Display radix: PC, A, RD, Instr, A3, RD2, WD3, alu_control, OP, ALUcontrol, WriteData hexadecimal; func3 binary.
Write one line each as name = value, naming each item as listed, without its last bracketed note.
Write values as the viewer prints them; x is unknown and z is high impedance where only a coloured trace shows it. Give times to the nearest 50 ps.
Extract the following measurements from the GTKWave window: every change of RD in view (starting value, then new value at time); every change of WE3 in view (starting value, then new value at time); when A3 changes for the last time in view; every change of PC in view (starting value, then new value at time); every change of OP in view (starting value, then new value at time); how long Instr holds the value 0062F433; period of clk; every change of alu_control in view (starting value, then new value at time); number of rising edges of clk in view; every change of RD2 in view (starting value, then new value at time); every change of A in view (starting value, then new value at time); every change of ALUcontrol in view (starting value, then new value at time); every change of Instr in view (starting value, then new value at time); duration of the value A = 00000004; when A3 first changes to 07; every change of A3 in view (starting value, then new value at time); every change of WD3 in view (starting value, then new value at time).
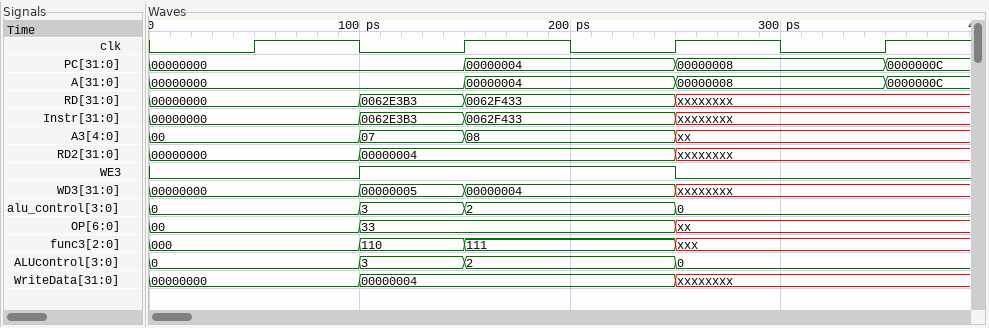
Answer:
every change of RD in view = 00000000, 0062E3B3 at 100 ps, 0062F433 at 150 ps, xxxxxxxx at 250 ps
every change of WE3 in view = 0, 1 at 100 ps, 0 at 250 ps
when A3 changes for the last time in view = 250 ps
every change of PC in view = 00000000, 00000004 at 150 ps, 00000008 at 250 ps, 0000000C at 350 ps
every change of OP in view = 00, 33 at 100 ps, xx at 250 ps
how long Instr holds the value 0062F433 = 100 ps
period of clk = 100 ps
every change of alu_control in view = 0, 3 at 100 ps, 2 at 150 ps, 0 at 250 ps
number of rising edges of clk in view = 4
every change of RD2 in view = 00000000, 00000004 at 100 ps, xxxxxxxx at 250 ps
every change of A in view = 00000000, 00000004 at 150 ps, 00000008 at 250 ps, 0000000C at 350 ps
every change of ALUcontrol in view = 0, 3 at 100 ps, 2 at 150 ps, 0 at 250 ps
every change of Instr in view = 00000000, 0062E3B3 at 100 ps, 0062F433 at 150 ps, xxxxxxxx at 250 ps
duration of the value A = 00000004 = 100 ps
when A3 first changes to 07 = 100 ps
every change of A3 in view = 00, 07 at 100 ps, 08 at 150 ps, xx at 250 ps
every change of WD3 in view = 00000000, 00000005 at 100 ps, 00000004 at 150 ps, xxxxxxxx at 250 ps
